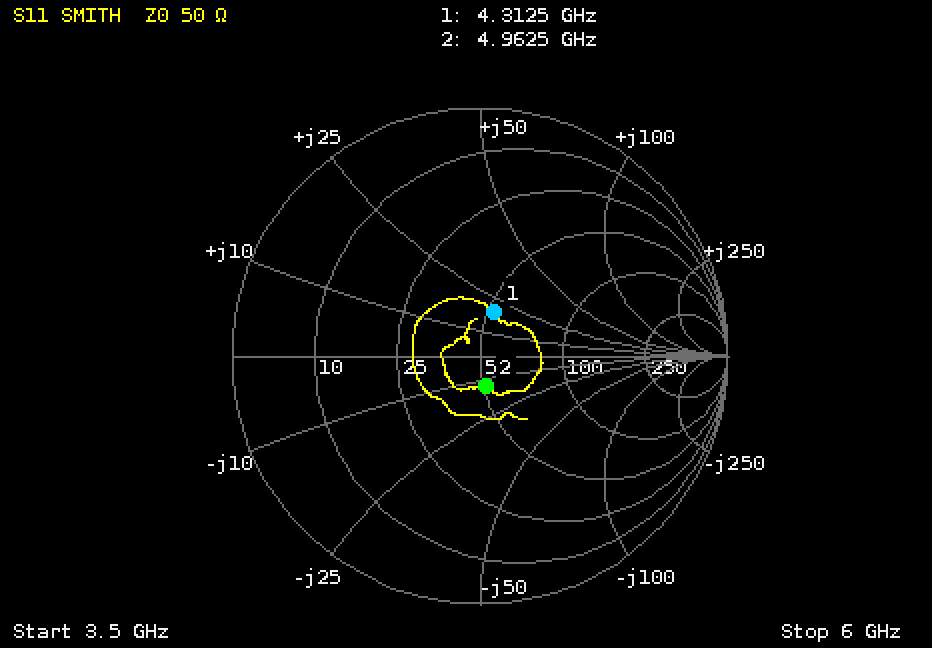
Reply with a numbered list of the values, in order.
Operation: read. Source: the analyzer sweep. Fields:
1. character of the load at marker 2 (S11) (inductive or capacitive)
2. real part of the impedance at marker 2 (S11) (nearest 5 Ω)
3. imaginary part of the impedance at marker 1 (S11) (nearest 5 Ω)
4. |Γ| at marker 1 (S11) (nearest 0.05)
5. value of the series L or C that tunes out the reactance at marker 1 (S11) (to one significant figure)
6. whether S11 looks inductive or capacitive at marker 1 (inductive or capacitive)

1. capacitive
2. 50 Ω
3. +20 Ω
4. 0.20
5. 2 pF
6. inductive
